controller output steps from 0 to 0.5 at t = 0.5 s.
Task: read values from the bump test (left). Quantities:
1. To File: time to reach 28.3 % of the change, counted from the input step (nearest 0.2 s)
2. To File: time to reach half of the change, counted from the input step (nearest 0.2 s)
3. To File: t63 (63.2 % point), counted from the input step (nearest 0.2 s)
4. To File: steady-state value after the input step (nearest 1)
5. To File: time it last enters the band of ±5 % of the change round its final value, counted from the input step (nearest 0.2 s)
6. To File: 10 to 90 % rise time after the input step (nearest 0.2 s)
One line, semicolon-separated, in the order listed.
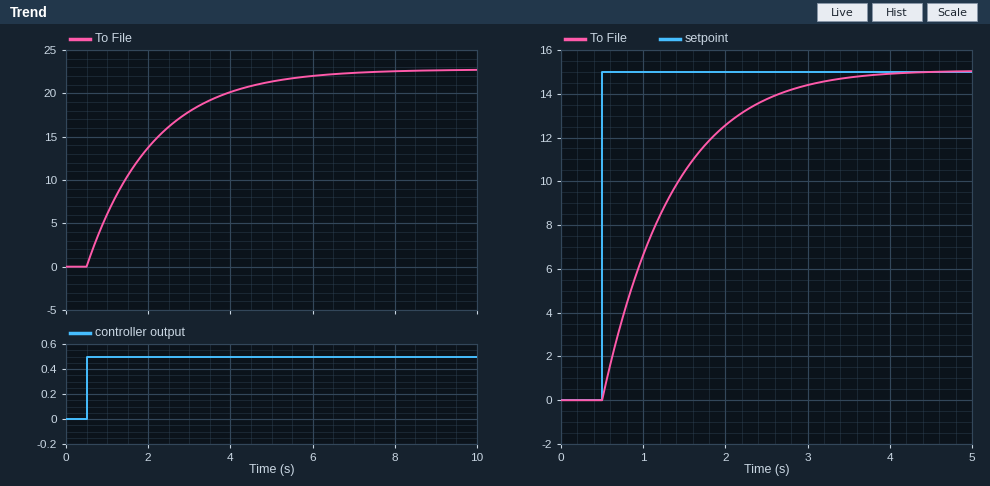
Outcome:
0.6 s; 1.2 s; 1.6 s; 23; 4.8 s; 3.6 s
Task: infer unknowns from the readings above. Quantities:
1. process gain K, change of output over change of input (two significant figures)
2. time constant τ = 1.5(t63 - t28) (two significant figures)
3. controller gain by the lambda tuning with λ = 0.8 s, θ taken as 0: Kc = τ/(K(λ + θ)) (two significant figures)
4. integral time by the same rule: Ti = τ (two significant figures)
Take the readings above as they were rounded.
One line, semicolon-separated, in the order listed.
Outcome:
46; 1.5 s; 0.041; 1.5 s
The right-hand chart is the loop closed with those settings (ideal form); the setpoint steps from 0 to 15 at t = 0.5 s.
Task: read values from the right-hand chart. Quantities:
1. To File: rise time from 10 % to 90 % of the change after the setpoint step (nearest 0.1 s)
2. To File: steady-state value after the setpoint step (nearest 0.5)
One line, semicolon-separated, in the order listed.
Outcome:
1.8 s; 15.0
